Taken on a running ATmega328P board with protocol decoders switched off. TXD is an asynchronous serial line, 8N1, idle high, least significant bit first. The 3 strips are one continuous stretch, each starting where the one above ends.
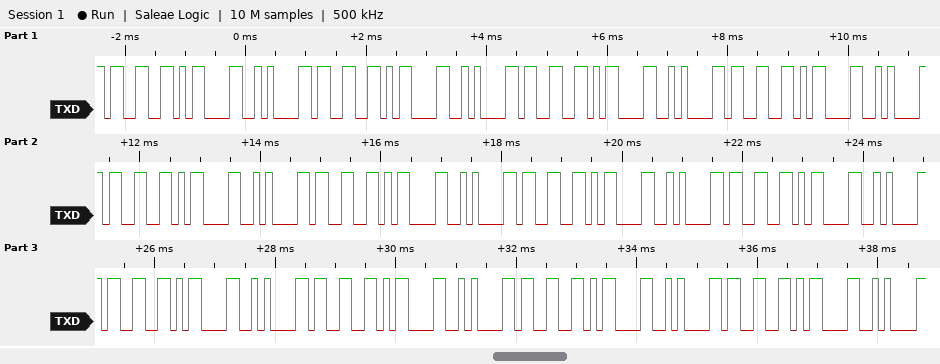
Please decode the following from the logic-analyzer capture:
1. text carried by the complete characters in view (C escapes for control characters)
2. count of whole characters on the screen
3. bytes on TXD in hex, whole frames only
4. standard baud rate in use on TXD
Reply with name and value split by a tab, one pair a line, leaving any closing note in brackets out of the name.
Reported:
text carried by the complete characters in view	"3\r\n3\r\n3\r\n3\r\n3\r\n3\r\n3\r\n3\r\n3\r\n3\r\n3\r\n3\r\n"
count of whole characters on the screen	36
bytes on TXD in hex, whole frames only	33 0D 0A 33 0D 0A 33 0D 0A 33 0D 0A 33 0D 0A 33 0D 0A 33 0D 0A 33 0D 0A 33 0D 0A 33 0D 0A 33 0D 0A 33 0D 0A
standard baud rate in use on TXD	9600 baud
